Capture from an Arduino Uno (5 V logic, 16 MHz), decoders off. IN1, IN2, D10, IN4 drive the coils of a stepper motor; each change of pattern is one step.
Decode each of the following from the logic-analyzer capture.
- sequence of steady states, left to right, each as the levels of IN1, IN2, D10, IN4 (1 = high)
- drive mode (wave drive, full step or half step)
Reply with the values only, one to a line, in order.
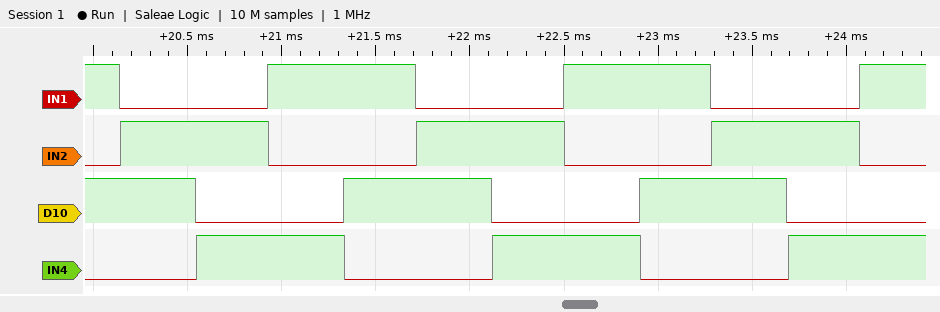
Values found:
1010 0110 0101 1001 1010 0110 0101 1001 1010 0110 0101 1001
full step
